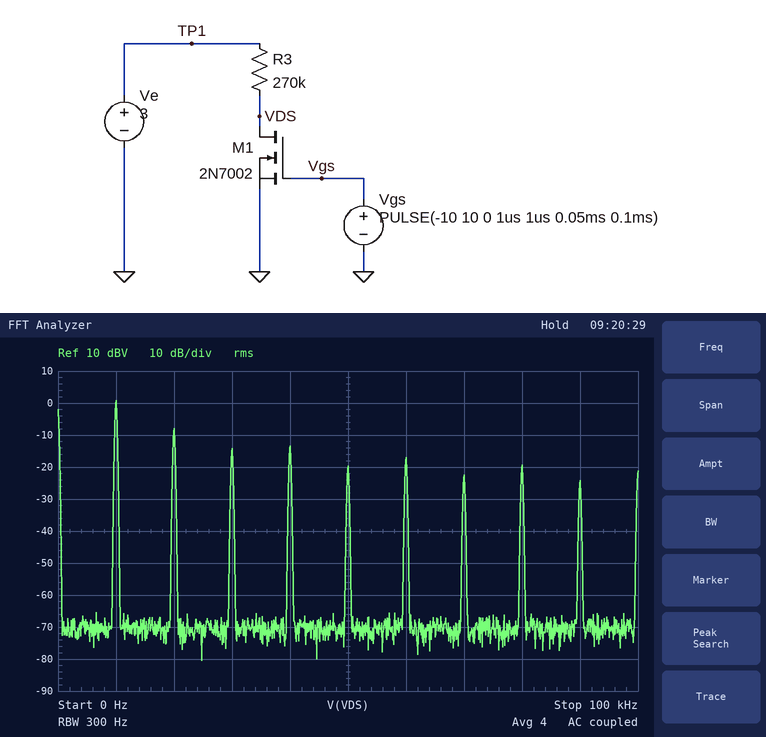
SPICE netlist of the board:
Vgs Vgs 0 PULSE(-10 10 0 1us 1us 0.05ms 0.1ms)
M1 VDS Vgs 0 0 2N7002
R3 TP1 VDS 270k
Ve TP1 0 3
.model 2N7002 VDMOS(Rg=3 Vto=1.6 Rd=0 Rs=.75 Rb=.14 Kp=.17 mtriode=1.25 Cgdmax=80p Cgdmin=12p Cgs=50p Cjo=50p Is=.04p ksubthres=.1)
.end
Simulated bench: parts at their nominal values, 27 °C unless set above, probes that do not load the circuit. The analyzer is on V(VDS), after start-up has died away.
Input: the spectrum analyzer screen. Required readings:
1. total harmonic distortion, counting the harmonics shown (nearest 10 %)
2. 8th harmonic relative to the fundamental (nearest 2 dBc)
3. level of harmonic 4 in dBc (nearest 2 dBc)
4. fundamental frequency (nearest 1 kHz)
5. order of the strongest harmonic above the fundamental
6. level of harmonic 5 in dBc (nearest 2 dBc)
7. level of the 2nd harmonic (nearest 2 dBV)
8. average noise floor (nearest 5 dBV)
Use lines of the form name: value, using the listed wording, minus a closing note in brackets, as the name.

total harmonic distortion, counting the harmonics shown: 50 %
8th harmonic relative to the fundamental: -20 dBc
level of harmonic 4 in dBc: -14 dBc
fundamental frequency: 10 kHz
order of the strongest harmonic above the fundamental: 2
level of harmonic 5 in dBc: -20 dBc
level of the 2nd harmonic: -8 dBV
average noise floor: -70 dBV
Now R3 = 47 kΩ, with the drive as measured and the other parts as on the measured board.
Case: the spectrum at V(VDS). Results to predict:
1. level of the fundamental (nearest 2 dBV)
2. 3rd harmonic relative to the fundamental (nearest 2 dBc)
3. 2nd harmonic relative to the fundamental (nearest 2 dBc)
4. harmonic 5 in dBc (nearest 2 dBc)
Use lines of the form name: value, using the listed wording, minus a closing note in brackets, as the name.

level of the fundamental: 2 dBV
3rd harmonic relative to the fundamental: -10 dBc
2nd harmonic relative to the fundamental: -18 dBc
harmonic 5 in dBc: -16 dBc
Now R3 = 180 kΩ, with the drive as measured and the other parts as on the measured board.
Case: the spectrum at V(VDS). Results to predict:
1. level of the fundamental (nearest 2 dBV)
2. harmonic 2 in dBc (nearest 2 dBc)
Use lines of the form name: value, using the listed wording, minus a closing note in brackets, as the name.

level of the fundamental: 2 dBV
harmonic 2 in dBc: -10 dBc
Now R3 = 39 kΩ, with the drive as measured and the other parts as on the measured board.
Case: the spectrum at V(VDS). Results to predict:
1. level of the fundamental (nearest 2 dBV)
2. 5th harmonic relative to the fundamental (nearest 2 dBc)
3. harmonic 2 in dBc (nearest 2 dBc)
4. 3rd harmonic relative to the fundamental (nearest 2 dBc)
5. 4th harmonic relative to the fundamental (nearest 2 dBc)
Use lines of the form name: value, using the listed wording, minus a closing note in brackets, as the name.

level of the fundamental: 2 dBV
5th harmonic relative to the fundamental: -16 dBc
harmonic 2 in dBc: -20 dBc
3rd harmonic relative to the fundamental: -10 dBc
4th harmonic relative to the fundamental: -20 dBc
